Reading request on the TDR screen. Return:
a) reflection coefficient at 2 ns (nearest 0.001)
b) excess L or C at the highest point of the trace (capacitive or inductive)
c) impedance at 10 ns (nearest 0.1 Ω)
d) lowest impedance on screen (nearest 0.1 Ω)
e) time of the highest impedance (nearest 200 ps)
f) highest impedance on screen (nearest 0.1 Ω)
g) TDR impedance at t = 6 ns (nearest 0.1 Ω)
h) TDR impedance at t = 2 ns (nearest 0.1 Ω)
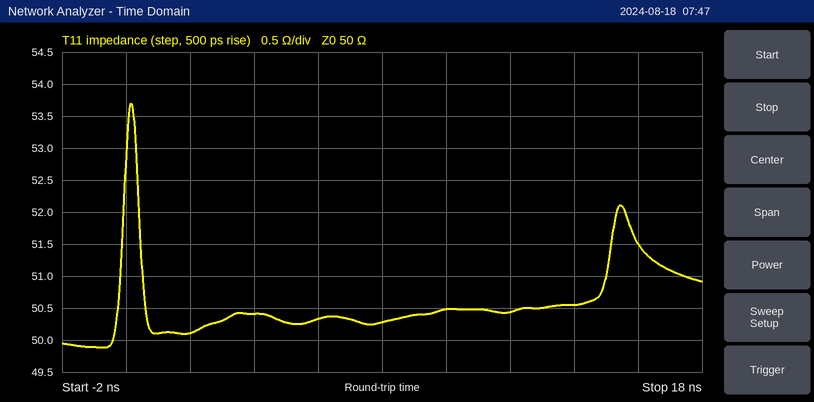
+0.001
inductive
50.5 Ω
49.9 Ω
200 ps
53.7 Ω
50.3 Ω
50.1 Ω
